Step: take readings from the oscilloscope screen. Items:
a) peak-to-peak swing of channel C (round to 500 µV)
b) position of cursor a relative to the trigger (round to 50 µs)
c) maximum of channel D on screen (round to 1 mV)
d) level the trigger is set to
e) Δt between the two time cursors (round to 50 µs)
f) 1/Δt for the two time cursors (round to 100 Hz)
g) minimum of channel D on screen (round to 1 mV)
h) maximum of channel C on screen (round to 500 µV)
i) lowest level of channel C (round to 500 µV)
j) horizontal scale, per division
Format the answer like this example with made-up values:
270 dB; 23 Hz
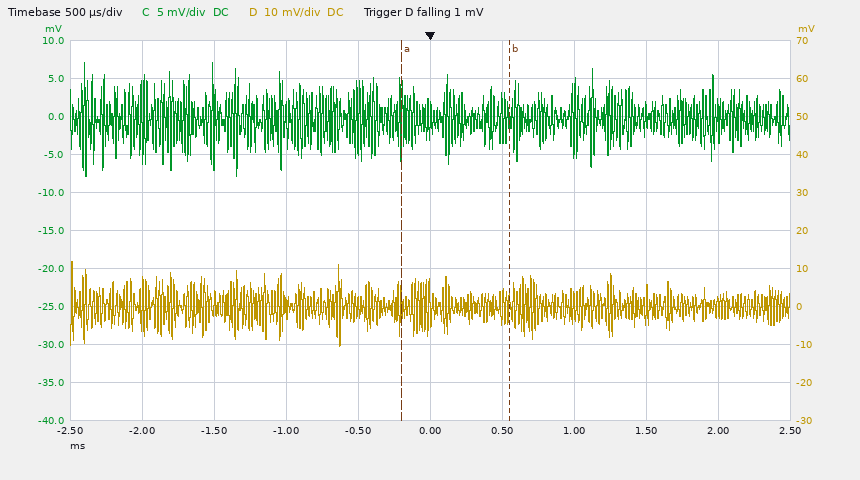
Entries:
15.0 mV; -200 µs; 12 mV; 1 mV; 750 µs; 1.3 kHz; -11 mV; 7.0 mV; -8.0 mV; 500 µs
